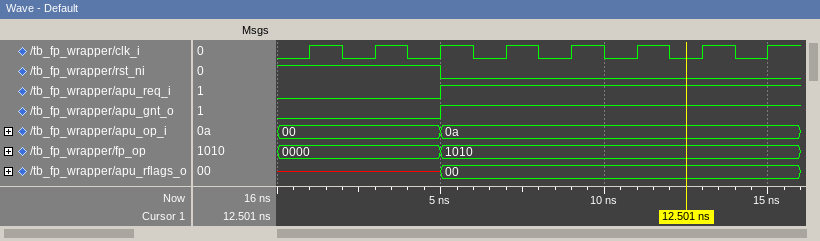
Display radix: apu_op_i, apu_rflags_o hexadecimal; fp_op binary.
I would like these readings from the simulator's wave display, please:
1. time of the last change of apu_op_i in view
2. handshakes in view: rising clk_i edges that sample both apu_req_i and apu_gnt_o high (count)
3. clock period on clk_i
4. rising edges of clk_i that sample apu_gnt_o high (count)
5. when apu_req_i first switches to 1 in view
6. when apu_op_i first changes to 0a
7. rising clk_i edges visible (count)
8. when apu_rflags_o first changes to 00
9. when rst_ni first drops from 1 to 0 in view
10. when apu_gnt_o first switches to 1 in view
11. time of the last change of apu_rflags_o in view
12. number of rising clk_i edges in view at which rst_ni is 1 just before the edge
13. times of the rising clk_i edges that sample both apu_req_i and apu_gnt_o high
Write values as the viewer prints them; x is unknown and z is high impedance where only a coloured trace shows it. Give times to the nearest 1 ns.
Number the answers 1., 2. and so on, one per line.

1. 5 ns
2. 5
3. 2 ns
4. 5
5. 5 ns
6. 5 ns
7. 8
8. 5 ns
9. 5 ns
10. 5 ns
11. 5 ns
12. 3
13. 7 ns, 9 ns, 11 ns, 13 ns, 15 ns
